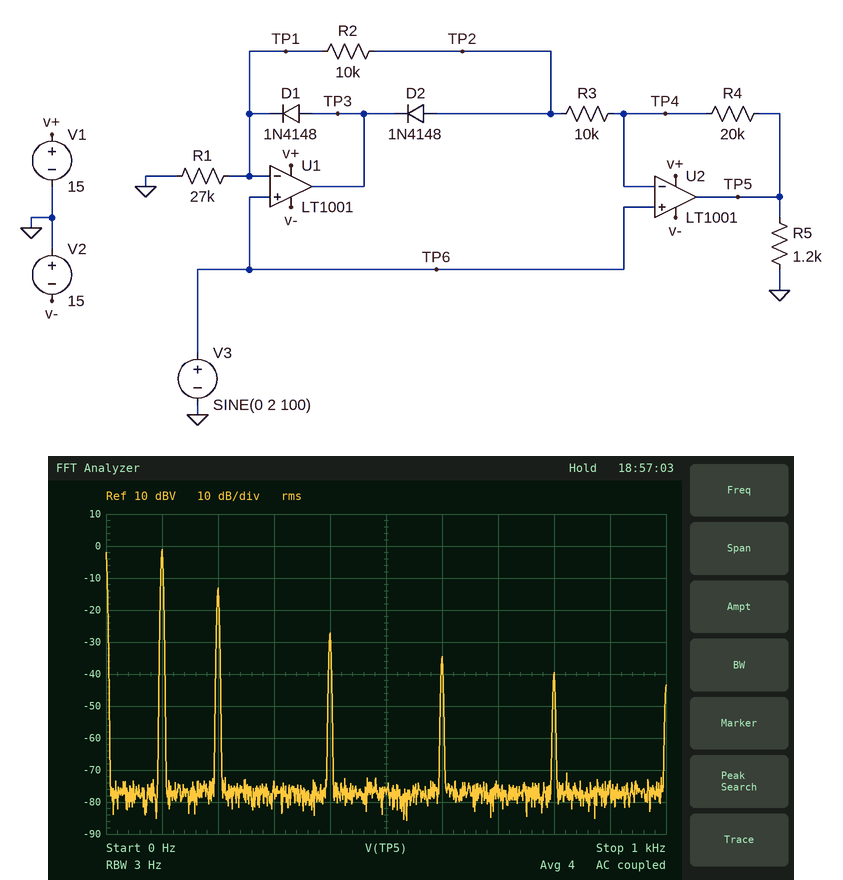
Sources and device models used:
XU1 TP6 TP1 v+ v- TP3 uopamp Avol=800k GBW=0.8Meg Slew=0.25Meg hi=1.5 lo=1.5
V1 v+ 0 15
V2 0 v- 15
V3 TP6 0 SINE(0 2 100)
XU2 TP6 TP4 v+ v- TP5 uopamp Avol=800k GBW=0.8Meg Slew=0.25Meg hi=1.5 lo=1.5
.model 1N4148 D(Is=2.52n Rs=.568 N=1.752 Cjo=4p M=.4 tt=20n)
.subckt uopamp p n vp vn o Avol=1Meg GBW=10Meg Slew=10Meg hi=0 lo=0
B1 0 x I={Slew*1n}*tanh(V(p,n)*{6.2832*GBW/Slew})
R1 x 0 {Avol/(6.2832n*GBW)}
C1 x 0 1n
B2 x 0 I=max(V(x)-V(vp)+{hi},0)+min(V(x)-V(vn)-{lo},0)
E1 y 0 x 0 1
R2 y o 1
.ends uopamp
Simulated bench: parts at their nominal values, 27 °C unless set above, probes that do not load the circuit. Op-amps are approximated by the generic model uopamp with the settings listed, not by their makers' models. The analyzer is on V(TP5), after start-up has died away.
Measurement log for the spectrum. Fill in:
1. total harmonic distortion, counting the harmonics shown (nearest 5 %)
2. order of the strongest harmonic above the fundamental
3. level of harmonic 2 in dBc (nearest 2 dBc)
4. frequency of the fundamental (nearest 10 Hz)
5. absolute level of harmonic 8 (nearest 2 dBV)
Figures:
25 %
2
-12 dBc
100 Hz
-40 dBV
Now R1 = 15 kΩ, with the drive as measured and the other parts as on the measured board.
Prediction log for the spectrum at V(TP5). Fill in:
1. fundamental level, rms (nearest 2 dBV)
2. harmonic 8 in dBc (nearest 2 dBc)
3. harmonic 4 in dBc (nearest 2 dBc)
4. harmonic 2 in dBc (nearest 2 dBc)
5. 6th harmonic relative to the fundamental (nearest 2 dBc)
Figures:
-6 dBV
-28 dBc
-16 dBc
-2 dBc
-22 dBc
